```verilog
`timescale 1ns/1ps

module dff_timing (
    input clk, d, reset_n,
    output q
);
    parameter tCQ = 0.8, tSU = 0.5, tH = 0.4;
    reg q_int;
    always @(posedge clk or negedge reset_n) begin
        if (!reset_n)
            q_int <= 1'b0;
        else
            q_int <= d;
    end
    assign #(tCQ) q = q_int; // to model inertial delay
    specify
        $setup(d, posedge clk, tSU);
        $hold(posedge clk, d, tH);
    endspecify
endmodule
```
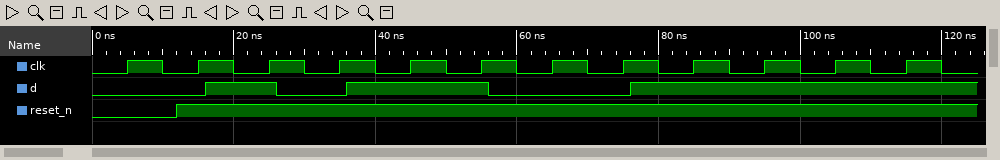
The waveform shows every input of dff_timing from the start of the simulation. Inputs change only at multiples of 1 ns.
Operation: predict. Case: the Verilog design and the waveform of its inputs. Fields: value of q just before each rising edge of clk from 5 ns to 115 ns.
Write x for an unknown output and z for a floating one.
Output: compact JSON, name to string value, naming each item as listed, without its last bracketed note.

{"value of q just before each rising edge of clk from 5 ns to 115 ns": "0 0 0 1 0 1 1 0 0 1 1 1"}
